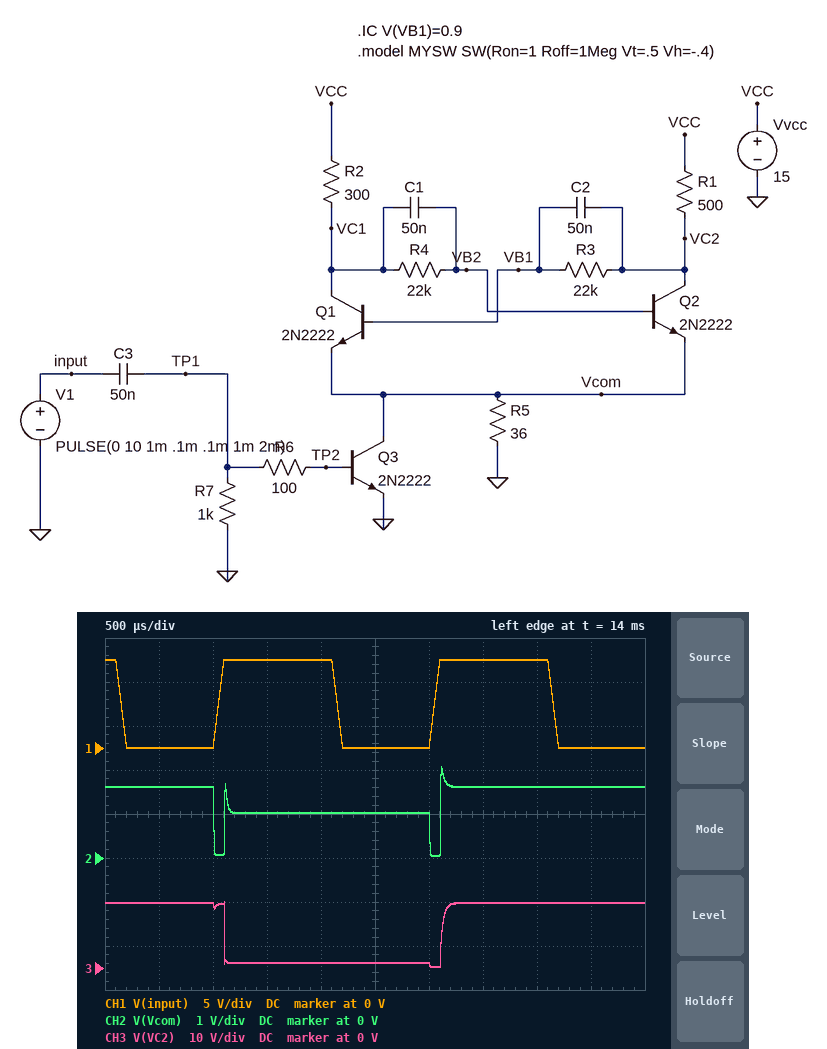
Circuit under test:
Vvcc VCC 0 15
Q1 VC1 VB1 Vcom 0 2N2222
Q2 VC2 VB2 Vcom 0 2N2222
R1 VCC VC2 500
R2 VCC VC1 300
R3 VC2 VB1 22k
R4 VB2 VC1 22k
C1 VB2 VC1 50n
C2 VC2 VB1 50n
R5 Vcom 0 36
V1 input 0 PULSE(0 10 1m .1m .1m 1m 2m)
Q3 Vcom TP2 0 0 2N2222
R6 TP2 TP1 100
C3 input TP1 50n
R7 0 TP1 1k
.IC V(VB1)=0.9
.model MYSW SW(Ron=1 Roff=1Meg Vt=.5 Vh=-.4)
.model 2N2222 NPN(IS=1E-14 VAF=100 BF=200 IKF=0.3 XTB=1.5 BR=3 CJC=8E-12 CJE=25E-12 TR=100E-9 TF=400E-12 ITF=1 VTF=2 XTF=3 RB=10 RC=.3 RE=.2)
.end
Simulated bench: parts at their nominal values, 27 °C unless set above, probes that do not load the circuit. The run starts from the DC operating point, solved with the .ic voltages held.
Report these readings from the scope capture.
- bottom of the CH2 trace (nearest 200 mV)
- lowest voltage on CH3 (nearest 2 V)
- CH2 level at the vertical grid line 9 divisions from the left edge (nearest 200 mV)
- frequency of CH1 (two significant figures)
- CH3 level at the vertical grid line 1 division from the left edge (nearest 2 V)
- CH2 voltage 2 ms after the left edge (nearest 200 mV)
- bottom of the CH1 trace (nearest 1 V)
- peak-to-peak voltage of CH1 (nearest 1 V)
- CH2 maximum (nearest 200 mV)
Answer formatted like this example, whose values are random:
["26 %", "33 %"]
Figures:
["0 V", "0 V", "1.6 V", "500 Hz", "14 V", "1.0 V", "0 V", "10 V", "2.0 V"]
